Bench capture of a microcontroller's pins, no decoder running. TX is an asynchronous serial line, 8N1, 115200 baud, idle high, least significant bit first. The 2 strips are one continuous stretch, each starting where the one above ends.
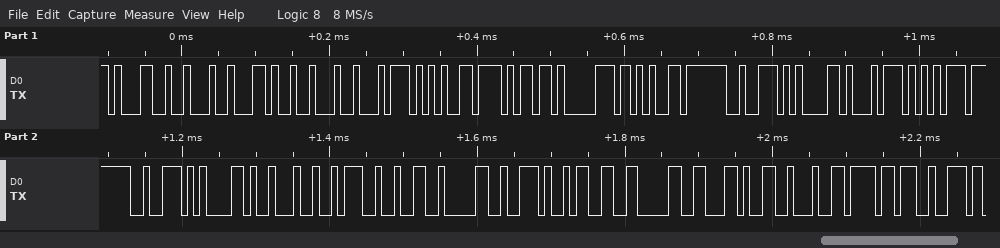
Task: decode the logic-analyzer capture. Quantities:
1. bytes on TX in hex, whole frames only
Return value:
31 22 2C 22 74 65 6D 70 65 72 61 74 75 72 61 22 3A 32 30 2E 33 30 2C 22 6F 72
